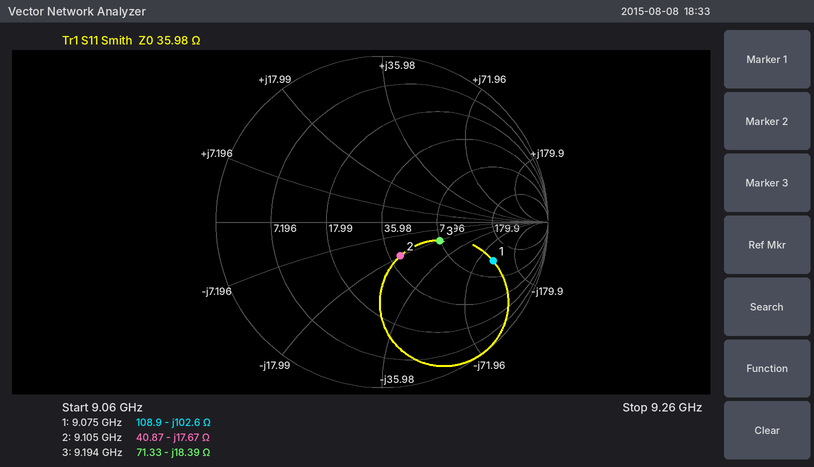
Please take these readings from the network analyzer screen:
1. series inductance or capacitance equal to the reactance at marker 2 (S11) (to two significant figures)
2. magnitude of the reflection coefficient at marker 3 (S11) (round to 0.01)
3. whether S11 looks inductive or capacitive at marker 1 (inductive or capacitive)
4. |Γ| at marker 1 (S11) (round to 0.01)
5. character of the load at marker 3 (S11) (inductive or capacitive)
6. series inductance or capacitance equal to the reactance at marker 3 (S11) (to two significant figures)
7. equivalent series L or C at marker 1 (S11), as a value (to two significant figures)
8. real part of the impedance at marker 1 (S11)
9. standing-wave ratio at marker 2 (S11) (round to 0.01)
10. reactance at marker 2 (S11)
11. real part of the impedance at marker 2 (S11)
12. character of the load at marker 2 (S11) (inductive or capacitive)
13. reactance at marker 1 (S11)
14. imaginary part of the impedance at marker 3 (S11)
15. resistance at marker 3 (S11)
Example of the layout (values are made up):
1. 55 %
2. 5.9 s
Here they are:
1. 990 fF
2. 0.37
3. capacitive
4. 0.71
5. capacitive
6. 940 fF
7. 170 fF
8. 108.9 Ω
9. 1.61
10. -17.67 Ω
11. 40.87 Ω
12. capacitive
13. -102.6 Ω
14. -18.39 Ω
15. 71.33 Ω
